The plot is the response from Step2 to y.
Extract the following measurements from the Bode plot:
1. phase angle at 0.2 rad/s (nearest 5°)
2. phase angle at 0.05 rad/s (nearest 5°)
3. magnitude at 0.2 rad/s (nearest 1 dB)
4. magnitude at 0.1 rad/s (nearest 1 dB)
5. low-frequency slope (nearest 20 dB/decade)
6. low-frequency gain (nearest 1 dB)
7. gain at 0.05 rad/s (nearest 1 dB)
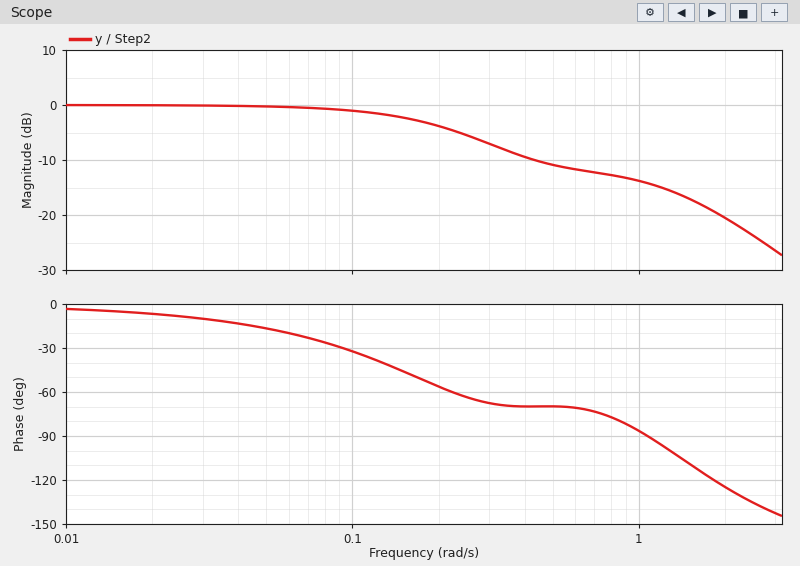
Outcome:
-55°
-15°
-4 dB
-1 dB
0 dB/decade
0 dB
0 dB
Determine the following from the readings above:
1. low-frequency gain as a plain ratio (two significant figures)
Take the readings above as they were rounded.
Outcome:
1.0
